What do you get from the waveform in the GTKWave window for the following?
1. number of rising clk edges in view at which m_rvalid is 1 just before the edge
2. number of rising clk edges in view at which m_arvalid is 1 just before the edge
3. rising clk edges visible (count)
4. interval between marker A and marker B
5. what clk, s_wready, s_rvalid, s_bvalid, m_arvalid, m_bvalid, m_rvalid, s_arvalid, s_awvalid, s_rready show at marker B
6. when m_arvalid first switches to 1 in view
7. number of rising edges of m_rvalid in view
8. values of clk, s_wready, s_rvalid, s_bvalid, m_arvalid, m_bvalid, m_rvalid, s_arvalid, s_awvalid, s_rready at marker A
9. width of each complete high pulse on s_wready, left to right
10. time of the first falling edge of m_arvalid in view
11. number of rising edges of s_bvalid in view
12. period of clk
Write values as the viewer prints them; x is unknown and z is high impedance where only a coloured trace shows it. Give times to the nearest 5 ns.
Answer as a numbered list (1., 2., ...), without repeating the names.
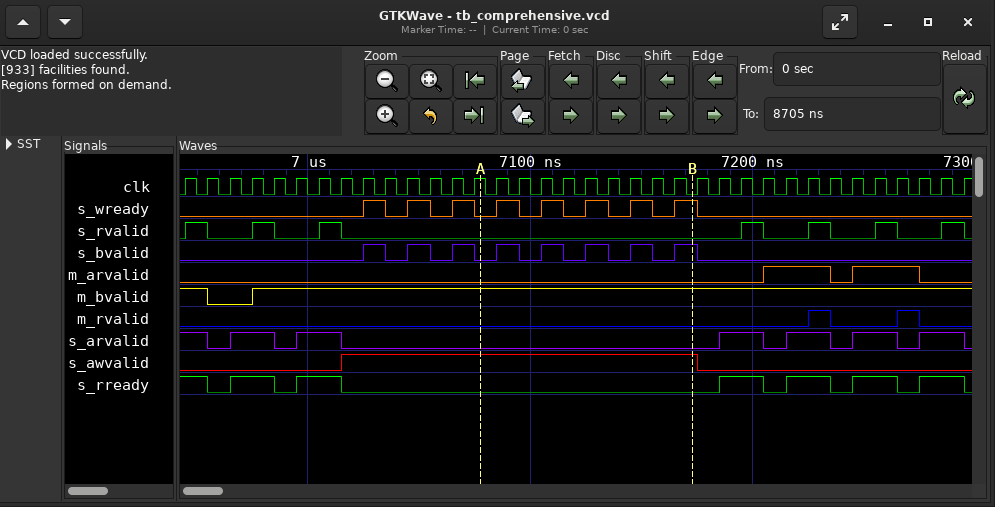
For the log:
1. 2
2. 6
3. 36
4. 95 ns
5. clk=0, s_wready=1, s_rvalid=0, s_bvalid=1, m_arvalid=0, m_bvalid=1, m_rvalid=0, s_arvalid=0, s_awvalid=1, s_rready=0
6. 7205 ns
7. 2
8. clk=1, s_wready=0, s_rvalid=0, s_bvalid=0, m_arvalid=0, m_bvalid=1, m_rvalid=0, s_arvalid=0, s_awvalid=1, s_rready=0
9. 10 ns, 10 ns, 10 ns, 10 ns, 10 ns, 10 ns, 10 ns, 10 ns
10. 7235 ns
11. 8
12. 10 ns
